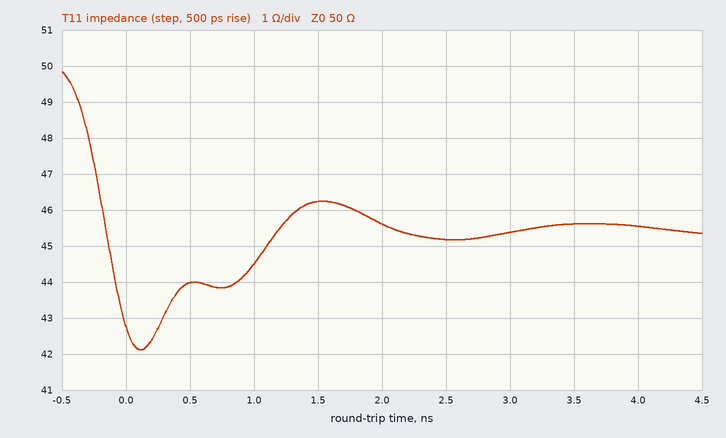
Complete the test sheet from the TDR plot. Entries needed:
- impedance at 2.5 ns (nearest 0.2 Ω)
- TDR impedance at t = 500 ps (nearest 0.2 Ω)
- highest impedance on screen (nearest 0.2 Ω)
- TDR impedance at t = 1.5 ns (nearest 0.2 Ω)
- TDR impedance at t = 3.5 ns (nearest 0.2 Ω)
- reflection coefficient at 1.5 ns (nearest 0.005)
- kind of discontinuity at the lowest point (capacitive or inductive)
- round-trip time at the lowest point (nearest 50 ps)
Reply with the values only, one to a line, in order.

45.2 Ω
44.0 Ω
49.8 Ω
46.2 Ω
45.6 Ω
-0.040
capacitive
100 ps
